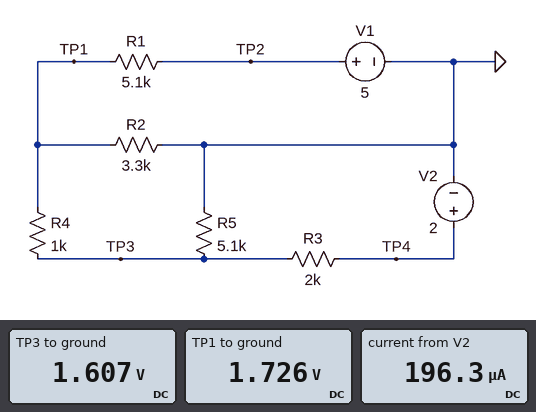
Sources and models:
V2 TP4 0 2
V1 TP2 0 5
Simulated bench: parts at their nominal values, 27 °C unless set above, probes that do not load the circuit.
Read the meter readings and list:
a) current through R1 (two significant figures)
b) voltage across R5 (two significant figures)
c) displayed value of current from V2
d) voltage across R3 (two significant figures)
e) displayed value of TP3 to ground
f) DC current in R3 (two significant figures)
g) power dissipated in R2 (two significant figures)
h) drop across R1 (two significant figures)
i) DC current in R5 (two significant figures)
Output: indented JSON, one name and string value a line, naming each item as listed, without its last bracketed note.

{
  "current through R1": "640 µA",
  "voltage across R5": "1.6 V",
  "displayed value of current from V2": "196.3 µA",
  "voltage across R3": "390 mV",
  "displayed value of TP3 to ground": "1.607 V",
  "DC current in R3": "200 µA",
  "power dissipated in R2": "900 µW",
  "drop across R1": "3.3 V",
  "DC current in R5": "320 µA"
}
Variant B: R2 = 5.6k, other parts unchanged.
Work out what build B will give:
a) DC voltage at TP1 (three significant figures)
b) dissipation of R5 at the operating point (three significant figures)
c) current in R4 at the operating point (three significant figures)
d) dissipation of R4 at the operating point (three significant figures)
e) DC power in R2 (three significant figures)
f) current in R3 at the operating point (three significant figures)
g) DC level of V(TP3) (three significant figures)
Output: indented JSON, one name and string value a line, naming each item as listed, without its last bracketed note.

{
  "DC voltage at TP1": "2.00 V",
  "dissipation of R5 at the operating point": "613 µW",
  "current in R4 at the operating point": "231 µA",
  "dissipation of R4 at the operating point": "53.4 µW",
  "DC power in R2": "714 µW",
  "current in R3 at the operating point": "116 µA",
  "DC level of V(TP3)": "1.77 V"
}
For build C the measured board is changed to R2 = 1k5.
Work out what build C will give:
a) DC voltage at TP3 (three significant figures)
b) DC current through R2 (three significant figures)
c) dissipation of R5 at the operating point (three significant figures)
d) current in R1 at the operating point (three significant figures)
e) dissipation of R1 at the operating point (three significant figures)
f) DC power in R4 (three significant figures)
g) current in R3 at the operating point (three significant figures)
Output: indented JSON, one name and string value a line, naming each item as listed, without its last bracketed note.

{
  "DC voltage at TP3": "1.32 V",
  "DC current through R2": "822 µA",
  "dissipation of R5 at the operating point": "340 µW",
  "current in R1 at the operating point": "739 µA",
  "dissipation of R1 at the operating point": "2.78 mW",
  "DC power in R4": "6.97 µW",
  "current in R3 at the operating point": "342 µA"
}
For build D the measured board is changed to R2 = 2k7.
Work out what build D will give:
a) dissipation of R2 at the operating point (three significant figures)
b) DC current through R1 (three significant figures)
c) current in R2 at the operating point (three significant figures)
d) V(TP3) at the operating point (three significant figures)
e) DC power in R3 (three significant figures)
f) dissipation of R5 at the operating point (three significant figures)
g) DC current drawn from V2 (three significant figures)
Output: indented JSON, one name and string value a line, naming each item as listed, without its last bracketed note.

{
  "dissipation of R2 at the operating point": "957 µW",
  "DC current through R1": "665 µA",
  "current in R2 at the operating point": "595 µA",
  "V(TP3) at the operating point": "1.54 V",
  "DC power in R3": "107 µW",
  "dissipation of R5 at the operating point": "463 µW",
  "DC current drawn from V2": "231 µA"
}
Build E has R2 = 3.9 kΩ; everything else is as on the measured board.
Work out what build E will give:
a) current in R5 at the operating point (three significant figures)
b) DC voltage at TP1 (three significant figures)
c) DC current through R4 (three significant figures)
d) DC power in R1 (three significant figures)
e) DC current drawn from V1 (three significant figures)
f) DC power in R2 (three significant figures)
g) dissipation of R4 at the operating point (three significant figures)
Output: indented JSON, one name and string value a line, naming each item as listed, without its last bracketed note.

{
  "current in R5 at the operating point": "326 µA",
  "DC voltage at TP1": "1.82 V",
  "DC current through R4": "157 µA",
  "DC power in R1": "1.98 mW",
  "DC current drawn from V1": "624 µA",
  "DC power in R2": "849 µW",
  "dissipation of R4 at the operating point": "24.7 µW"
}
